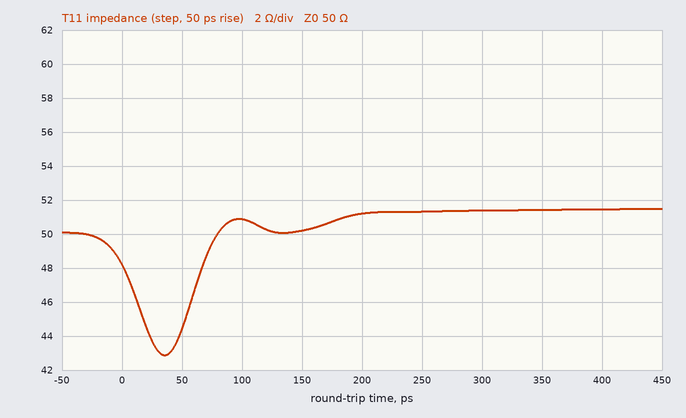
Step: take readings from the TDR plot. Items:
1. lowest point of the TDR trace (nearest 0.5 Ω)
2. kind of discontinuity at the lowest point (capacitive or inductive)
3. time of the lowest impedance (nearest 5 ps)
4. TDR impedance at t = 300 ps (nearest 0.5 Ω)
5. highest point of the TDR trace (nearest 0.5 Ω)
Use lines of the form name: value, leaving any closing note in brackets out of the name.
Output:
lowest point of the TDR trace: 43.0 Ω
kind of discontinuity at the lowest point: capacitive
time of the lowest impedance: 35 ps
TDR impedance at t = 300 ps: 51.5 Ω
highest point of the TDR trace: 51.5 Ω
